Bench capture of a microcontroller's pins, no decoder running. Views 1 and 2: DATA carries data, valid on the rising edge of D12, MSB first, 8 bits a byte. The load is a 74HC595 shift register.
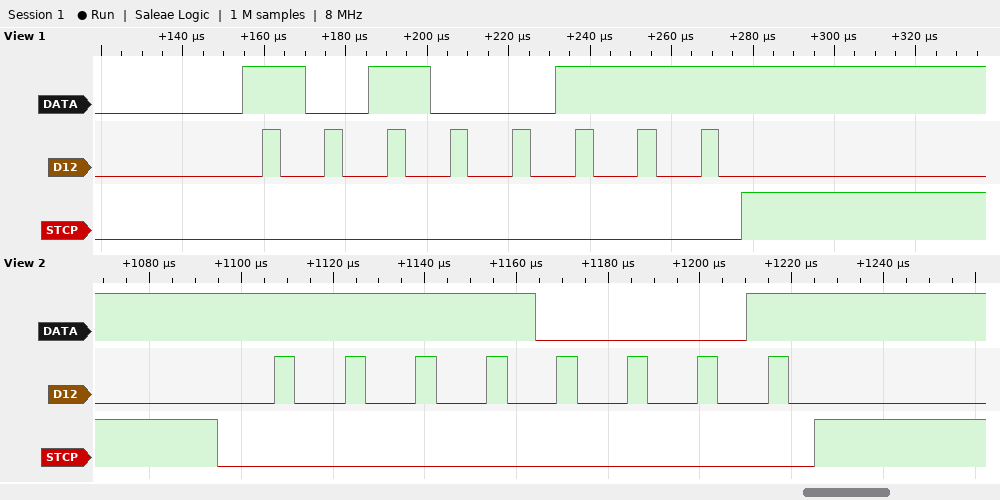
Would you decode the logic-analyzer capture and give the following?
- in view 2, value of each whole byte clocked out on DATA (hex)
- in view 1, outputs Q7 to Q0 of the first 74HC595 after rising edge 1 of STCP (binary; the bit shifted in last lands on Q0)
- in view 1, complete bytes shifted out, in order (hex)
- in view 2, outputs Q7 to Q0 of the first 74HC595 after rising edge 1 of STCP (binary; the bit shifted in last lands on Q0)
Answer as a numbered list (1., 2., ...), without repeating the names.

1. F1
2. 10100111
3. 0xA7
4. 11110001
